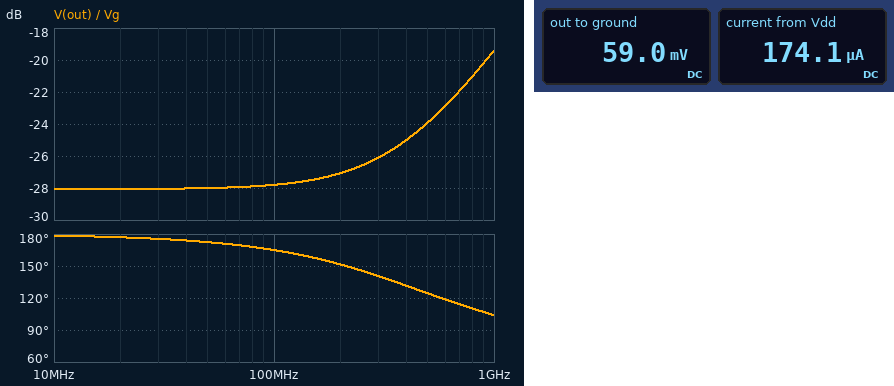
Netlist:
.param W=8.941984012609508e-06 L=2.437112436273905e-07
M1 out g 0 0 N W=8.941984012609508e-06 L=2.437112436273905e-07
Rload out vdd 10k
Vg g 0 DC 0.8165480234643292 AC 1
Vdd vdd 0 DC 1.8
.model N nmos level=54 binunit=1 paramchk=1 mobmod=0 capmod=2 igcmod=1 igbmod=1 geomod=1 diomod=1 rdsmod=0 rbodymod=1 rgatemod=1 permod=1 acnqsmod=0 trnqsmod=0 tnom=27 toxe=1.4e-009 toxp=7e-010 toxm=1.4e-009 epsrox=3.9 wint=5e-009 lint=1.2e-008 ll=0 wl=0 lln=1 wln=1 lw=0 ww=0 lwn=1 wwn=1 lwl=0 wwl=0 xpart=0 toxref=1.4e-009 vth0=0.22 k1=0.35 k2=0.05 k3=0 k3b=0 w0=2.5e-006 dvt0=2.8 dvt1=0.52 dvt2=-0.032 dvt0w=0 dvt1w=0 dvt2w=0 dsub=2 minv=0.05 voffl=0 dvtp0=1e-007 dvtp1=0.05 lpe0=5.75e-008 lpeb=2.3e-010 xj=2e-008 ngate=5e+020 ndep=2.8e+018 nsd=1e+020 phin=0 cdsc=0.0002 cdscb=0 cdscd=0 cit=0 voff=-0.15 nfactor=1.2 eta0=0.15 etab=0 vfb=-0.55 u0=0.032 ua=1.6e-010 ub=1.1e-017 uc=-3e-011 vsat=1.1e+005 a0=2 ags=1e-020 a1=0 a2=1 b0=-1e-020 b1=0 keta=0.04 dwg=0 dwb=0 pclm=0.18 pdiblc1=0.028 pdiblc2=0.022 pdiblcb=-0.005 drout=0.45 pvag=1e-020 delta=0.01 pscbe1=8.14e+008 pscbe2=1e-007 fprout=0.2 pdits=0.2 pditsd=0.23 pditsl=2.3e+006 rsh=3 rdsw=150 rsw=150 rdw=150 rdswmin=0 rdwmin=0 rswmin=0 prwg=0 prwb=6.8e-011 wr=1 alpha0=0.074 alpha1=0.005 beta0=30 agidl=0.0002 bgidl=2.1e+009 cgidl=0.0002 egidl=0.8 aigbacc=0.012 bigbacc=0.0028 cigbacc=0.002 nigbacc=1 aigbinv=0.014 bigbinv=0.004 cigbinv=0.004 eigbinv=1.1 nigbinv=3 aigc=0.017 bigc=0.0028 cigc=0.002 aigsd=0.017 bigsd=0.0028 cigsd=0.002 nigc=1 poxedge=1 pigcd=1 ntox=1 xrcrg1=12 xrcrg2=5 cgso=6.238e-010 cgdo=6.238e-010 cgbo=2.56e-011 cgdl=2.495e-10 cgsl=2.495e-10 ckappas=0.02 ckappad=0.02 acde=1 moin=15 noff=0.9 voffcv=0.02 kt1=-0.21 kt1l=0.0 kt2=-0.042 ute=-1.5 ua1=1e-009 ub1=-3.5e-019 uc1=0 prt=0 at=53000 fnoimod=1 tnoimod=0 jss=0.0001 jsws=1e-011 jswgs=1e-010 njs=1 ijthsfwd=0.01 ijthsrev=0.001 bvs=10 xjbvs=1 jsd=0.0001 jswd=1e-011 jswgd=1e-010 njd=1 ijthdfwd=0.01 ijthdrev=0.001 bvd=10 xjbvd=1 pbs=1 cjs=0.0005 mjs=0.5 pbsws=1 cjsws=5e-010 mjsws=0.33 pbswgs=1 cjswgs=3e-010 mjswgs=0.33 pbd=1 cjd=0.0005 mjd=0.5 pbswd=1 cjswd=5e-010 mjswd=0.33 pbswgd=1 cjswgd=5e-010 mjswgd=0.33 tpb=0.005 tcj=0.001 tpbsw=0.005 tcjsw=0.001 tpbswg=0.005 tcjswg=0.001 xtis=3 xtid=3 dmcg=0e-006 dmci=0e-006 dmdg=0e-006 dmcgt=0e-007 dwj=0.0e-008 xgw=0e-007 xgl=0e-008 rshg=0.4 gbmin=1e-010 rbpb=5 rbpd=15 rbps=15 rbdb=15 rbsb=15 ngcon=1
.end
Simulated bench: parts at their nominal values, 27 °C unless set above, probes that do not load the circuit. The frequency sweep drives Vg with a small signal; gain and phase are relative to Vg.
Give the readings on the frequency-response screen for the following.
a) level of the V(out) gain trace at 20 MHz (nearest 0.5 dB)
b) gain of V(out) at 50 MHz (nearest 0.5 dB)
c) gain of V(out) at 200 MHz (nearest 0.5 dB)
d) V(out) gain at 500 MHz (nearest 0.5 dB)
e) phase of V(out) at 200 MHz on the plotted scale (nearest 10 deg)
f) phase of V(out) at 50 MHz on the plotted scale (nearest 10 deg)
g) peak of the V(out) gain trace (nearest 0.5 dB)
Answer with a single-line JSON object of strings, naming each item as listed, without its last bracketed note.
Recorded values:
{"level of the V(out) gain trace at 20 MHz": "-28.0 dB", "gain of V(out) at 50 MHz": "-28.0 dB", "gain of V(out) at 200 MHz": "-27.0 dB", "V(out) gain at 500 MHz": "-24.0 dB", "phase of V(out) at 200 MHz on the plotted scale": "150 deg", "phase of V(out) at 50 MHz on the plotted scale": "170 deg", "peak of the V(out) gain trace": "-19.5 dB"}
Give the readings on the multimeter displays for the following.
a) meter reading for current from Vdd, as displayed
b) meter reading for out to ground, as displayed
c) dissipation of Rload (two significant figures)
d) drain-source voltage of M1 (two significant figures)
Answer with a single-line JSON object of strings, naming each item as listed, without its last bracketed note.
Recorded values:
{"meter reading for current from Vdd, as displayed": "174.1 µA", "meter reading for out to ground, as displayed": "59.0 mV", "dissipation of Rload": "300 µW", "drain-source voltage of M1": "59 mV"}
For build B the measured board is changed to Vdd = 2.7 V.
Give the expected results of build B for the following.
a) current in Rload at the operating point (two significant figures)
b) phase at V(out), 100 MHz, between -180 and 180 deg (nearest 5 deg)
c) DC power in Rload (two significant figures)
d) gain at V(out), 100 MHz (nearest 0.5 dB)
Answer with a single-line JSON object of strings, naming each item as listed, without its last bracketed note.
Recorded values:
{"current in Rload at the operating point": "260 µA", "phase at V(out), 100 MHz, between -180 and 180 deg": "170 deg", "DC power in Rload": "680 µW", "gain at V(out), 100 MHz": "-22.5 dB"}
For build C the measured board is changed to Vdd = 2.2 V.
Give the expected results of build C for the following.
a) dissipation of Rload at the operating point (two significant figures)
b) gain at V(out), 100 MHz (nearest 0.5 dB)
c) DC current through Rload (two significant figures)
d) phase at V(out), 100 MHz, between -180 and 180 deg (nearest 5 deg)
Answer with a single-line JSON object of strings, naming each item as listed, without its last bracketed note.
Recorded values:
{"dissipation of Rload at the operating point": "450 µW", "gain at V(out), 100 MHz": "-25.5 dB", "DC current through Rload": "210 µA", "phase at V(out), 100 MHz, between -180 and 180 deg": "170 deg"}
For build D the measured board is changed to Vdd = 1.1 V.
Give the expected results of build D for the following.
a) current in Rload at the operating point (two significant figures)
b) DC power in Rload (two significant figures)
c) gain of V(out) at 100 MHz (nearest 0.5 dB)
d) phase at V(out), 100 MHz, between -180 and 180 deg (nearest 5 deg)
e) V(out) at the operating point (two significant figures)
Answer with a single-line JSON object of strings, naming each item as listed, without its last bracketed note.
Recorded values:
{"current in Rload at the operating point": "110 µA", "DC power in Rload": "110 µW", "gain of V(out) at 100 MHz": "-33.0 dB", "phase at V(out), 100 MHz, between -180 and 180 deg": "155 deg", "V(out) at the operating point": "35 mV"}
